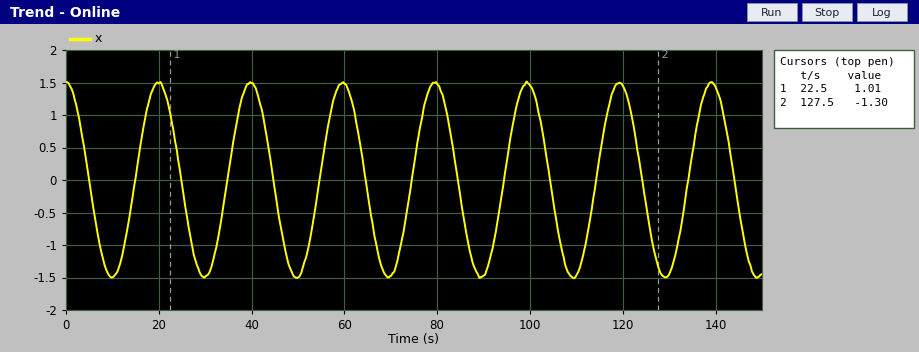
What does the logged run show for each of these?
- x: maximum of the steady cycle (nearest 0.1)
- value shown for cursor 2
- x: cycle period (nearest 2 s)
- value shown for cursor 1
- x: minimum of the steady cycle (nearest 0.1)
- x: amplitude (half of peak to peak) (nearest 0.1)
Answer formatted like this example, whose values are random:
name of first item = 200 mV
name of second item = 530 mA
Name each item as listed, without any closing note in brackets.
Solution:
x: maximum of the steady cycle = 1.5
value shown for cursor 2 = -1.30
x: cycle period = 20 s
value shown for cursor 1 = 1.01
x: minimum of the steady cycle = -1.5
x: amplitude (half of peak to peak) = 1.5
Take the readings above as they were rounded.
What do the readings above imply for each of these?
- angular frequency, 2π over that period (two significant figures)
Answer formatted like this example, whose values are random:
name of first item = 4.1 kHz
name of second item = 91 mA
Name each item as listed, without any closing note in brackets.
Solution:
angular frequency, 2π over that period = 0.31 rad/s
